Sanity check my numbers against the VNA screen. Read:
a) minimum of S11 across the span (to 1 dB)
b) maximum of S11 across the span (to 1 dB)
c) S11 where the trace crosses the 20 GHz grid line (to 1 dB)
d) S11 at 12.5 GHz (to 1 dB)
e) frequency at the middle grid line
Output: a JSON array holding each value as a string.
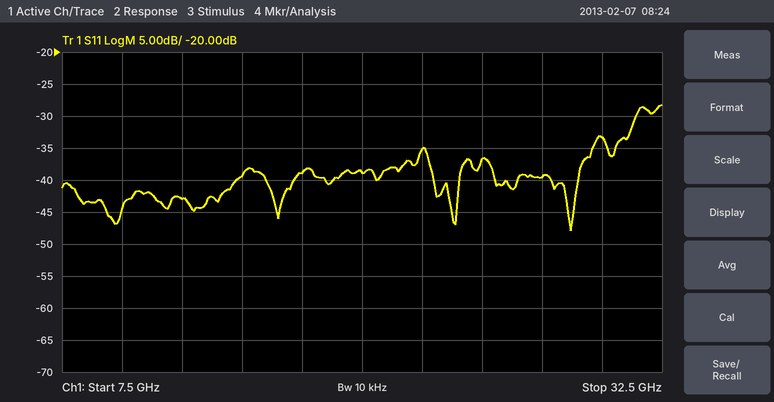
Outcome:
["-48 dB", "-28 dB", "-39 dB", "-43 dB", "20 GHz"]
